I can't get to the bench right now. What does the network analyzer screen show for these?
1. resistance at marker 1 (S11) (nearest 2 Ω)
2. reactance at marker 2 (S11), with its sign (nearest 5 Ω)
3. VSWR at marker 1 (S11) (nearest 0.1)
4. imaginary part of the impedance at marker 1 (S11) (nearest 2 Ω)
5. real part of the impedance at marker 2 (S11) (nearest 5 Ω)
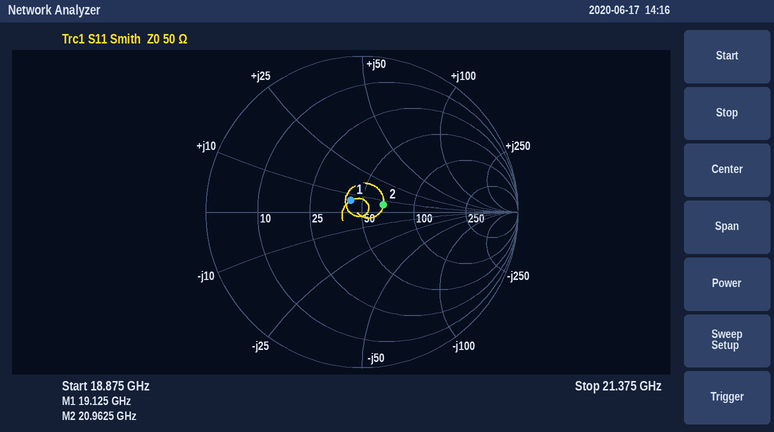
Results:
42 Ω
+5 Ω
1.2
+6 Ω
65 Ω
